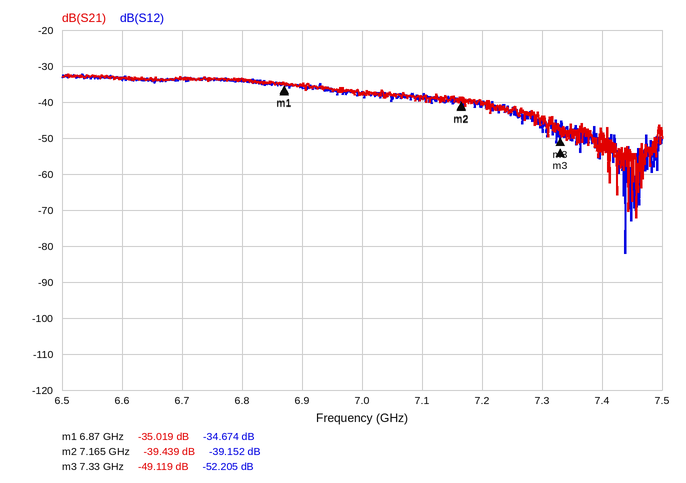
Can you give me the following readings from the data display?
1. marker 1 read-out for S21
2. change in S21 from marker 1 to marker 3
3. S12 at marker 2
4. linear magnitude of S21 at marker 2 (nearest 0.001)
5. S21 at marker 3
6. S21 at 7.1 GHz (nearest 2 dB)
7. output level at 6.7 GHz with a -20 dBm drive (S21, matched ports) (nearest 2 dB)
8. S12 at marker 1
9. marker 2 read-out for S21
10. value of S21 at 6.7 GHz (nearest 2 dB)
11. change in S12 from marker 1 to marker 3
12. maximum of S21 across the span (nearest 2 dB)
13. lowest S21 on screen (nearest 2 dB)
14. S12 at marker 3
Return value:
-35.019 dB
-14.100 dB
-39.152 dB
0.011
-49.119 dB
-38 dB
-54 dBm
-34.674 dB
-39.439 dB
-34 dB
-17.531 dB
-32 dB
-72 dB
-52.205 dB
